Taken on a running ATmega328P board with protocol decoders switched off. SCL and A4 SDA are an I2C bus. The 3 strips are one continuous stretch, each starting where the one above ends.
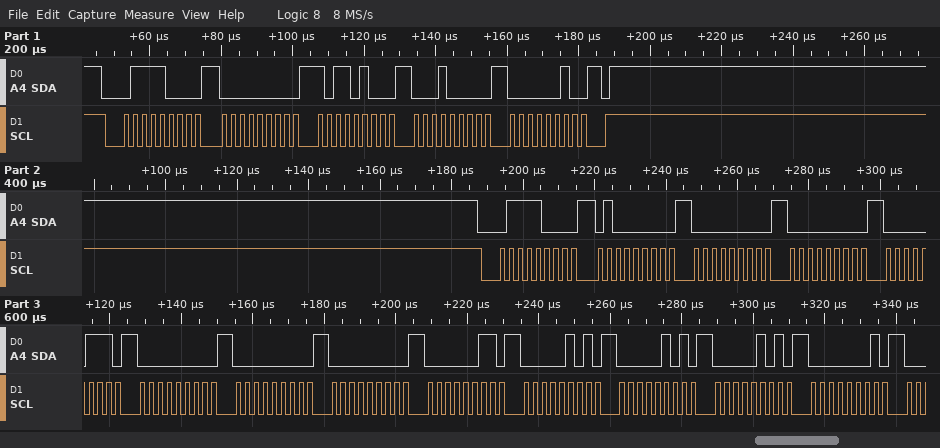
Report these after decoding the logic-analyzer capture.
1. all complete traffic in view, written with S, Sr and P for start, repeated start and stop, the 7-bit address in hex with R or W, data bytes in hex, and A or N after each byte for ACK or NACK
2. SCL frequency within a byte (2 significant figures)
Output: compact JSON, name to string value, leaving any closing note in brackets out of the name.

{"all complete traffic in view, written with S, Sr and P for start, repeated start and stop, the 7-bit address in hex with R or W, data bytes in hex, and A or N after each byte for ACK or NACK": "S 3CW A 00 A B4 A 10 A 02 A P S 3CW A 40 A 00 A 00 A 07 A 00 A 00 A 00 A 03 A 05 A 05 A 05 A 01 A", "SCL frequency within a byte": "400 kHz"}
